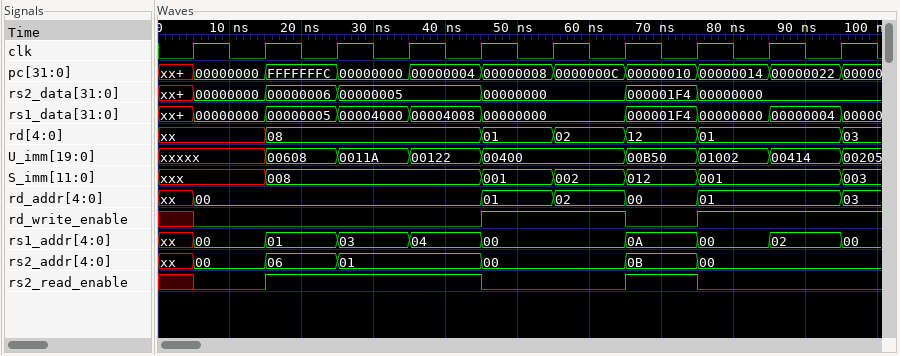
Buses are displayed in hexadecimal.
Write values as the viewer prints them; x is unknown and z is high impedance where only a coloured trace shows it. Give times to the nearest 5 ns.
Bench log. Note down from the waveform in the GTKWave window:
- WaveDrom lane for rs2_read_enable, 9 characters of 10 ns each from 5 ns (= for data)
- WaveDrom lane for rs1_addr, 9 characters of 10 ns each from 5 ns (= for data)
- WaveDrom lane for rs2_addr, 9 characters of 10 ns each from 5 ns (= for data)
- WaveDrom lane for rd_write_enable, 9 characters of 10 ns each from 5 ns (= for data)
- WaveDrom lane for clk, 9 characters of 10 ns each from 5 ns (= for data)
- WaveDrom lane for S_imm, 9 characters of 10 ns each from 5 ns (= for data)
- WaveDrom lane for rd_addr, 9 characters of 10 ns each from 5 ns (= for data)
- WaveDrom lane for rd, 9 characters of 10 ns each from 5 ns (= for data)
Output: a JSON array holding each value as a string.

["{name: 'rs2_read_enable', wave: '01..0.10.'}", "{name: 'rs1_addr', wave: '=====.===', data: '00 01 03 04 00 0A 00 02'}", "{name: 'rs2_addr', wave: '===.=.==.', data: '00 06 01 00 0B 00'}", "{name: 'rd_write_enable', wave: '0...1.01.'}", "{name: 'clk', wave: 'p........'}", "{name: 'S_imm', wave: 'x=..====.', data: '008 001 002 012 001'}", "{name: 'rd_addr', wave: '=...====.', data: '00 01 02 00 01'}", "{name: 'rd', wave: 'x=..====.', data: '08 01 02 12 01'}"]
